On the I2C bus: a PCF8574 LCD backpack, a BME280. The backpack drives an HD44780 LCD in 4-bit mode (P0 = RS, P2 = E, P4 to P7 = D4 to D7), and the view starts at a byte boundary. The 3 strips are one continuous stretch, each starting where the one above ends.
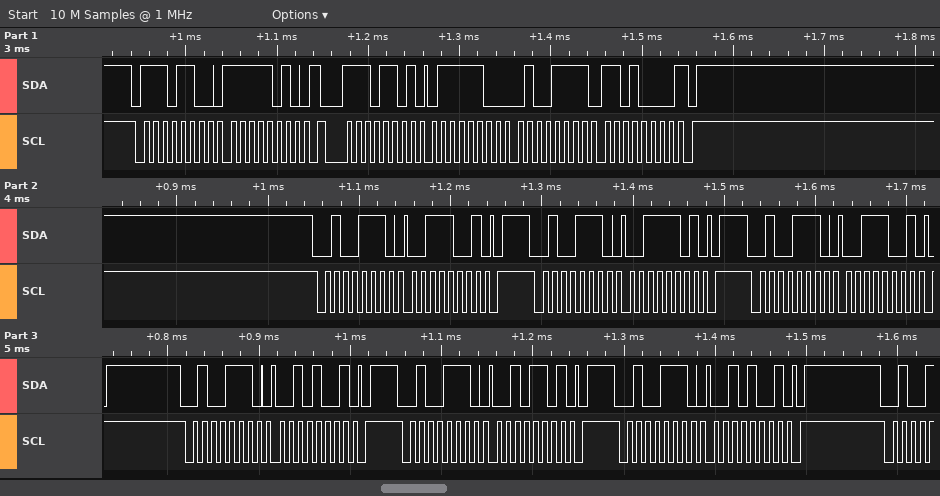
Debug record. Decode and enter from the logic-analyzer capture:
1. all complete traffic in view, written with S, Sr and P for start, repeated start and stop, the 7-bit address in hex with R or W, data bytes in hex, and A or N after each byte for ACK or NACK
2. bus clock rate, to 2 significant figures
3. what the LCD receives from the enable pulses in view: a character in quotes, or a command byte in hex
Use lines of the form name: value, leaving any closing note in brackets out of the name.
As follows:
all complete traffic in view, written with S, Sr and P for start, repeated start and stop, the 7-bit address in hex with R or W, data bytes in hex, and A or N after each byte for ACK or NACK: S 76W A FA A Sr 76R A 7C A 4F A D0 N P S 27W A 39 A P S 27W A 3D A P S 27W A 39 A P S 27W A 29 A P S 27W A 2D A P S 27W A 29 A P
bus clock rate, to 2 significant figures: 100 kHz
what the LCD receives from the enable pulses in view: a character in quotes, or a command byte in hex: '2'
